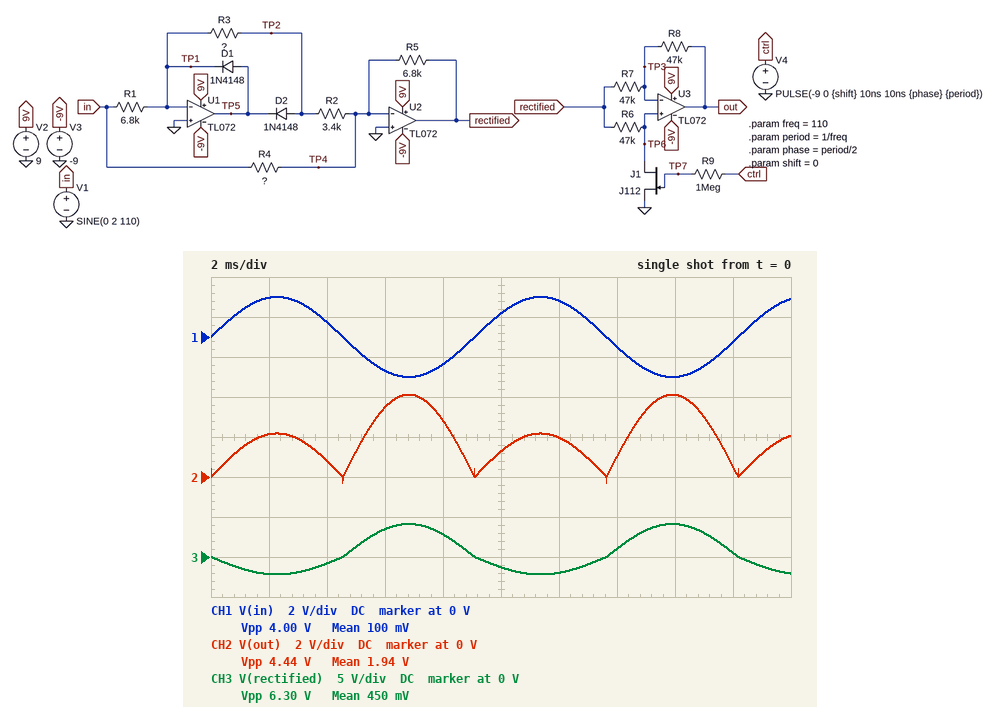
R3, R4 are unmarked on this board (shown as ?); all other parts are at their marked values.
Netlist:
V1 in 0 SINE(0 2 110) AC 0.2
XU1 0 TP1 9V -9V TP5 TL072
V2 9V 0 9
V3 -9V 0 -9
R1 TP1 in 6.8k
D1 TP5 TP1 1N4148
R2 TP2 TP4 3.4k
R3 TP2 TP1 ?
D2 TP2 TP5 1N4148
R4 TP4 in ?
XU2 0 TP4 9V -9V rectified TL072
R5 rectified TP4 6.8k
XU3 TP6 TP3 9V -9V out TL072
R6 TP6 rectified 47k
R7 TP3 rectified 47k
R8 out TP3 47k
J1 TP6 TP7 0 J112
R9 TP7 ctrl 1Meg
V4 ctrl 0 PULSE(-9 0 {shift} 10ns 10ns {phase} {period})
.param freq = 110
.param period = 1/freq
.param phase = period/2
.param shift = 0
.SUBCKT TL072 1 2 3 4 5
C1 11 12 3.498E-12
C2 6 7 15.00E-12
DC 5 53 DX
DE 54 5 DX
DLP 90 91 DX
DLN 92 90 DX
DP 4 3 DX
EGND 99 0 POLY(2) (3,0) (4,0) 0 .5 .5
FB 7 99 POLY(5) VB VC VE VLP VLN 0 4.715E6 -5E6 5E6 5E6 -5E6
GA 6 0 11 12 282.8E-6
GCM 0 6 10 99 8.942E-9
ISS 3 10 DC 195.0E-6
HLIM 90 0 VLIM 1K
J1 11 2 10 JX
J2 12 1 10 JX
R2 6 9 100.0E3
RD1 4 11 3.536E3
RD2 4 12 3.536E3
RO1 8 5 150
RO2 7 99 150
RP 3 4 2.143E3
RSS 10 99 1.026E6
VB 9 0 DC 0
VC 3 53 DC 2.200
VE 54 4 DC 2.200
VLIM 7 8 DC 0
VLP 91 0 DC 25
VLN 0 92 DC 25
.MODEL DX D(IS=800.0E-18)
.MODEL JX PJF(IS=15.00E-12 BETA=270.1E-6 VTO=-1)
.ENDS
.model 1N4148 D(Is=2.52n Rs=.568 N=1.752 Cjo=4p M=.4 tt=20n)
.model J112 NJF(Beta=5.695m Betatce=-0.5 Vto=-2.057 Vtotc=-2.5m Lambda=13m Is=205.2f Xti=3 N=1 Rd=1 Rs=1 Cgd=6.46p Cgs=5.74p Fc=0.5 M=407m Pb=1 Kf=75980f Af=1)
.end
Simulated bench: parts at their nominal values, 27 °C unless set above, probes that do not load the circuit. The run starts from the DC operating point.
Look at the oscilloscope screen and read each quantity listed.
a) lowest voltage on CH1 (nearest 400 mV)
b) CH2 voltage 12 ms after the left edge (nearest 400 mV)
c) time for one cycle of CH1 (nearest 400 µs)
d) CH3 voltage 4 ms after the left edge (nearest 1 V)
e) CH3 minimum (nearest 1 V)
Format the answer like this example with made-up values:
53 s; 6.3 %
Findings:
-2.0 V; 2.0 V; 9.2 ms; -1 V; -2 V
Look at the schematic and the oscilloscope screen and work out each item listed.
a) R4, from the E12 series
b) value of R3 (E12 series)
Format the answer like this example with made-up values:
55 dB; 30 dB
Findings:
3.3 kΩ; 3.3 kΩ
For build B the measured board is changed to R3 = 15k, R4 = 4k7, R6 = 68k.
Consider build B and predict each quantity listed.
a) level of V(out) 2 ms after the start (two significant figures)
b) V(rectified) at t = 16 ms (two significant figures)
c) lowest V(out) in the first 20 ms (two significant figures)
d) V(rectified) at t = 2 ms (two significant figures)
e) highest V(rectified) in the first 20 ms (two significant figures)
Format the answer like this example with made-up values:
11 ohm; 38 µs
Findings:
-5.8 V; 2.9 V; -5.9 V; 5.8 V; 5.9 V
